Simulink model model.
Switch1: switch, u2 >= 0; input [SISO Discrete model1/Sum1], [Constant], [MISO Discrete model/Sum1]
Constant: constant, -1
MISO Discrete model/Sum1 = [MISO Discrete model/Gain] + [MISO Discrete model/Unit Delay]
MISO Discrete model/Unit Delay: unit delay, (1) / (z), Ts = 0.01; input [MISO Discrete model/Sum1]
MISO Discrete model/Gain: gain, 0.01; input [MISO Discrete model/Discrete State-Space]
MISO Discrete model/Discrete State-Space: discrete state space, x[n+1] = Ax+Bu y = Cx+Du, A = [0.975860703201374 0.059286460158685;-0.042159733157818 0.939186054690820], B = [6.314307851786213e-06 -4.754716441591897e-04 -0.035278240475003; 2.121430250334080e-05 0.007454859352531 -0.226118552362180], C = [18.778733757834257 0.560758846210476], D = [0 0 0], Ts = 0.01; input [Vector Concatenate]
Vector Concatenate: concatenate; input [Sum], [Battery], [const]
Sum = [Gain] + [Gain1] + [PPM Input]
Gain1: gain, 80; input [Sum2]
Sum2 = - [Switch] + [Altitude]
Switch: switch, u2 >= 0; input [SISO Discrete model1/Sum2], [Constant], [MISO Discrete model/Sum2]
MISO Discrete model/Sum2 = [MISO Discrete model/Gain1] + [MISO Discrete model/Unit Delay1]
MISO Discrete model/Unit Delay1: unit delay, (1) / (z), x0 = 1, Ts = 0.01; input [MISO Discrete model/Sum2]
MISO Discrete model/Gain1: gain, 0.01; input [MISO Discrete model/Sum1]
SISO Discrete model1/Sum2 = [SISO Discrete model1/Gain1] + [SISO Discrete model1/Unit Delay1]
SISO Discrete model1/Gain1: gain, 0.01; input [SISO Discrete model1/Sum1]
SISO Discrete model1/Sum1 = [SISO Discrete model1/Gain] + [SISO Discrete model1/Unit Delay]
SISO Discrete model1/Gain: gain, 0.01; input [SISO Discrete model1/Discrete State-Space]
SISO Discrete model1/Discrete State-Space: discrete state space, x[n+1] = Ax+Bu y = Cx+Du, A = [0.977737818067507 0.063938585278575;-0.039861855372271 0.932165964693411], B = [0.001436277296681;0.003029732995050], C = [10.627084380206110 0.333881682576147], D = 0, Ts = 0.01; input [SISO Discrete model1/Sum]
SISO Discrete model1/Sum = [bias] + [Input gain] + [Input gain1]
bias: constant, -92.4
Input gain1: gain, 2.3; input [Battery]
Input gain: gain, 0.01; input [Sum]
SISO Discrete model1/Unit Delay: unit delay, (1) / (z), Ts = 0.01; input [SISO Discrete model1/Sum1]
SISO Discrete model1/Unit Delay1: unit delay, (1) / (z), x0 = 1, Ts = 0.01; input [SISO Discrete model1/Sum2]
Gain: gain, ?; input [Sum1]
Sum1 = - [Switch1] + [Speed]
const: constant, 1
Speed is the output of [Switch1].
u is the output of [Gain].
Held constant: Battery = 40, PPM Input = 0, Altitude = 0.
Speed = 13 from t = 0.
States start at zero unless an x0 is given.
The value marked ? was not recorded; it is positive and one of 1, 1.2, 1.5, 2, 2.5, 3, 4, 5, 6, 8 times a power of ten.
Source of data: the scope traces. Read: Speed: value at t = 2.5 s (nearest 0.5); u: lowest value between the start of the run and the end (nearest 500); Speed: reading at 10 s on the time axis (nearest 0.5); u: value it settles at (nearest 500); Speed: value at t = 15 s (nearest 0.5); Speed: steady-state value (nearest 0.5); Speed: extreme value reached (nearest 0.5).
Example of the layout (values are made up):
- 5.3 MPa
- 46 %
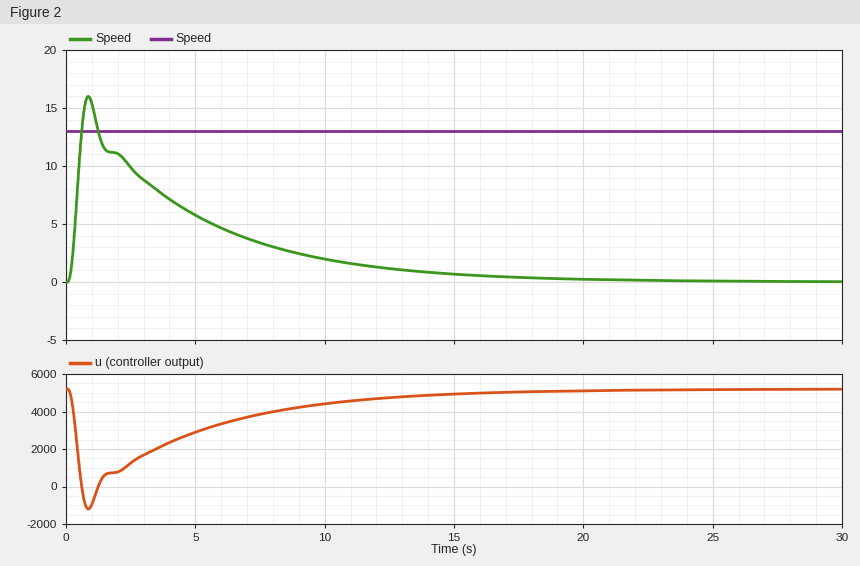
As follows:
- 10.0
- -1000
- 2.0
- 5000
- 0.5
- 0.0
- 16.0
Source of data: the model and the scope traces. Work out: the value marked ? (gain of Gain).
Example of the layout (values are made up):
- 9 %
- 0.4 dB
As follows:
- 400
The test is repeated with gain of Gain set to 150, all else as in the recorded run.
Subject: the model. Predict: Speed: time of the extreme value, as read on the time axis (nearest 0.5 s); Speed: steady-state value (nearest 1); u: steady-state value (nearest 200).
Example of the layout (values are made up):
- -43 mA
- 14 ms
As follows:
- 1.5 s
- 0
- 2000
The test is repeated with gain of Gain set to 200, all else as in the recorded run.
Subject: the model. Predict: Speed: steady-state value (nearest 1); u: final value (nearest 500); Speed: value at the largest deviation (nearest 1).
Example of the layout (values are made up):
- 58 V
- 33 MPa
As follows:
- 0
- 2500
- 13
